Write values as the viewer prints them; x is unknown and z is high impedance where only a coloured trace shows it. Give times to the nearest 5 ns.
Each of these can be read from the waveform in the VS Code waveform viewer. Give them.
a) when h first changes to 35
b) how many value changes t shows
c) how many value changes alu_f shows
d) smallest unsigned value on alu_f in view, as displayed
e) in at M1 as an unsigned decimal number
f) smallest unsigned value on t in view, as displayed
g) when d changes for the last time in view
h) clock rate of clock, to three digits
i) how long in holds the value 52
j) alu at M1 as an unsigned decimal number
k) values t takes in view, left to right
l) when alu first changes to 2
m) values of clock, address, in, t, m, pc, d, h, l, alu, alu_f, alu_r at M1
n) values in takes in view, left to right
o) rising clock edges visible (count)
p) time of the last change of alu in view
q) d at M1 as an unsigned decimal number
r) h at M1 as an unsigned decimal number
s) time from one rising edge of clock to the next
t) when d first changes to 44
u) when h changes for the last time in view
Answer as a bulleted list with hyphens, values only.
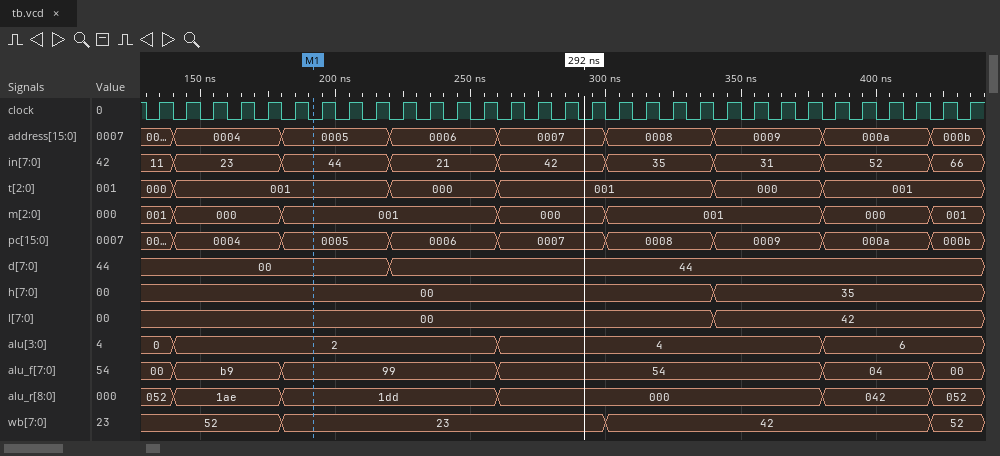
- 340 ns
- 5
- 5
- 00
- 68
- 000
- 220 ns
- 100 MHz
- 40 ns
- 2
- 000, 001, 000, 001, 000, 001
- 140 ns
- clock=0, address=0005, in=44, t=001, m=001, pc=0005, d=00, h=00, l=00, alu=2, alu_f=99, alu_r=1dd
- 11, 23, 44, 21, 42, 35, 31, 52, 66
- 31
- 380 ns
- 0
- 0
- 10 ns
- 220 ns
- 340 ns
